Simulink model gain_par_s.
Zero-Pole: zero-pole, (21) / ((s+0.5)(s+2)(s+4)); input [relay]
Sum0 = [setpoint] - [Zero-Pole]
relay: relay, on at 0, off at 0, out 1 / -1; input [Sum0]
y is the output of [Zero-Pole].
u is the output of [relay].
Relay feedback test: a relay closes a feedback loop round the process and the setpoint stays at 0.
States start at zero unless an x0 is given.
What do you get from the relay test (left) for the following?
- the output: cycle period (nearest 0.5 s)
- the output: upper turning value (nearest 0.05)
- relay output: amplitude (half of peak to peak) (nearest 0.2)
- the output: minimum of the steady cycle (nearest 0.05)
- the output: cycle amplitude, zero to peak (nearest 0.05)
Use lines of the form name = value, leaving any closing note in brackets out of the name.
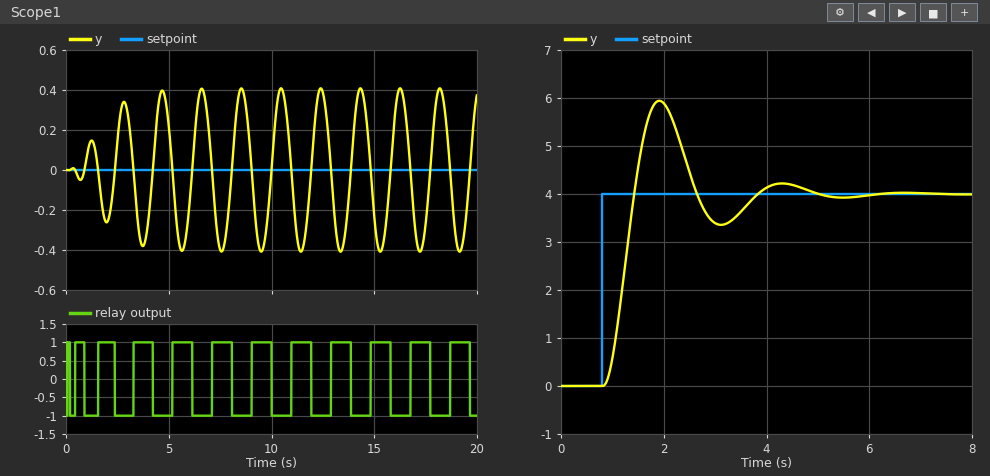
the output: cycle period = 2.0 s
the output: upper turning value = 0.40
relay output: amplitude (half of peak to peak) = 1.0
the output: minimum of the steady cycle = -0.40
the output: cycle amplitude, zero to peak = 0.40
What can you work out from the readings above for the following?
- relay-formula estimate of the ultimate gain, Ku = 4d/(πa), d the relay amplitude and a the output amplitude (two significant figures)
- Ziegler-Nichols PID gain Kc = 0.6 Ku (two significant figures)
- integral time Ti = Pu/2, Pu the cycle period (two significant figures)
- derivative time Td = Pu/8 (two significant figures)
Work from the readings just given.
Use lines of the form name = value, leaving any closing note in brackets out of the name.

relay-formula estimate of the ultimate gain, Ku = 4d/(πa), d the relay amplitude and a the output amplitude = 3.2
Ziegler-Nichols PID gain Kc = 0.6 Ku = 1.9
integral time Ti = Pu/2, Pu the cycle period = 1.0 s
derivative time Td = Pu/8 = 0.25 s
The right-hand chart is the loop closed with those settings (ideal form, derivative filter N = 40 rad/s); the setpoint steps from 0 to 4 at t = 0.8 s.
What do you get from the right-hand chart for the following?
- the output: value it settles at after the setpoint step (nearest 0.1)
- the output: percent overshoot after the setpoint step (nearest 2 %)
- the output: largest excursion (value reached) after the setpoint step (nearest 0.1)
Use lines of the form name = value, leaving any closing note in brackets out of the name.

the output: value it settles at after the setpoint step = 4.0
the output: percent overshoot after the setpoint step = 48 %
the output: largest excursion (value reached) after the setpoint step = 5.9
